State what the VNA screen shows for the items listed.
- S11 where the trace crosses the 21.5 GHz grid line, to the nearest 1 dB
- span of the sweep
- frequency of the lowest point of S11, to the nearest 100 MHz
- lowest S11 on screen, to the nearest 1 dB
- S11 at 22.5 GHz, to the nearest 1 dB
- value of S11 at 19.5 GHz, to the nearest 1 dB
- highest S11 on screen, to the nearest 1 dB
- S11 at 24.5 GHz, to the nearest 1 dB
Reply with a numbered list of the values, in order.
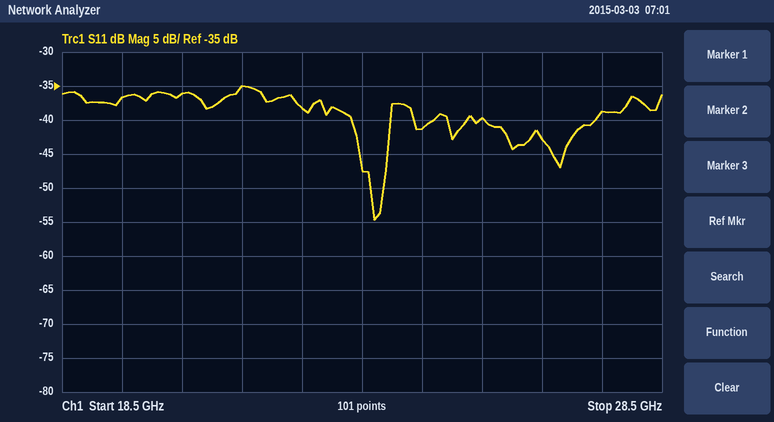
1. -35 dB
2. 10 GHz
3. 23.7 GHz
4. -55 dB
5. -38 dB
6. -37 dB
7. -35 dB
8. -41 dB
